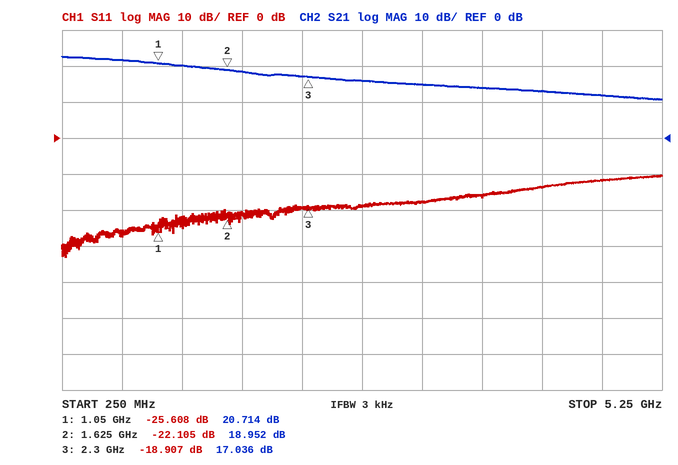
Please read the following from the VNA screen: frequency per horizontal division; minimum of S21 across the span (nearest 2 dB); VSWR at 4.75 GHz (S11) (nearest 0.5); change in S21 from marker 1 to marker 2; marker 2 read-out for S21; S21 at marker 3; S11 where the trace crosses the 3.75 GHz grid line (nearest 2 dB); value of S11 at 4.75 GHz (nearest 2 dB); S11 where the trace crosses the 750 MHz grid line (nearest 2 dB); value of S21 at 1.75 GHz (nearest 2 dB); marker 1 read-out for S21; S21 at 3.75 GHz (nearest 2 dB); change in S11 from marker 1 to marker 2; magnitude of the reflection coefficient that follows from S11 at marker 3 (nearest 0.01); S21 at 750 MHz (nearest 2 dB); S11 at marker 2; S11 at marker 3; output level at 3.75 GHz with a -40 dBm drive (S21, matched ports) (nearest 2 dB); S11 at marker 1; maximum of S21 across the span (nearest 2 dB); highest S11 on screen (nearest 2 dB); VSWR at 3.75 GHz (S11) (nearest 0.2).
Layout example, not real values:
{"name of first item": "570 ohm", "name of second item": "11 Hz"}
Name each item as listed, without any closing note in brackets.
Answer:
{"frequency per horizontal division": "500 MHz", "minimum of S21 across the span": "10 dB", "VSWR at 4.75 GHz (S11)": "1.5", "change in S21 from marker 1 to marker 2": "-1.762 dB", "marker 2 read-out for S21": "18.952 dB", "S21 at marker 3": "17.036 dB", "S11 where the trace crosses the 3.75 GHz grid line": "-16 dB", "value of S11 at 4.75 GHz": "-12 dB", "S11 where the trace crosses the 750 MHz grid line": "-26 dB", "value of S21 at 1.75 GHz": "18 dB", "marker 1 read-out for S21": "20.714 dB", "S21 at 3.75 GHz": "14 dB", "change in S11 from marker 1 to marker 2": "3.503 dB", "magnitude of the reflection coefficient that follows from S11 at marker 3": "0.11", "S21 at 750 MHz": "22 dB", "S11 at marker 2": "-22.105 dB", "S11 at marker 3": "-18.907 dB", "output level at 3.75 GHz with a -40 dBm drive (S21, matched ports)": "-26 dBm", "S11 at marker 1": "-25.608 dB", "maximum of S21 across the span": "22 dB", "highest S11 on screen": "-10 dB", "VSWR at 3.75 GHz (S11)": "1.4"}
